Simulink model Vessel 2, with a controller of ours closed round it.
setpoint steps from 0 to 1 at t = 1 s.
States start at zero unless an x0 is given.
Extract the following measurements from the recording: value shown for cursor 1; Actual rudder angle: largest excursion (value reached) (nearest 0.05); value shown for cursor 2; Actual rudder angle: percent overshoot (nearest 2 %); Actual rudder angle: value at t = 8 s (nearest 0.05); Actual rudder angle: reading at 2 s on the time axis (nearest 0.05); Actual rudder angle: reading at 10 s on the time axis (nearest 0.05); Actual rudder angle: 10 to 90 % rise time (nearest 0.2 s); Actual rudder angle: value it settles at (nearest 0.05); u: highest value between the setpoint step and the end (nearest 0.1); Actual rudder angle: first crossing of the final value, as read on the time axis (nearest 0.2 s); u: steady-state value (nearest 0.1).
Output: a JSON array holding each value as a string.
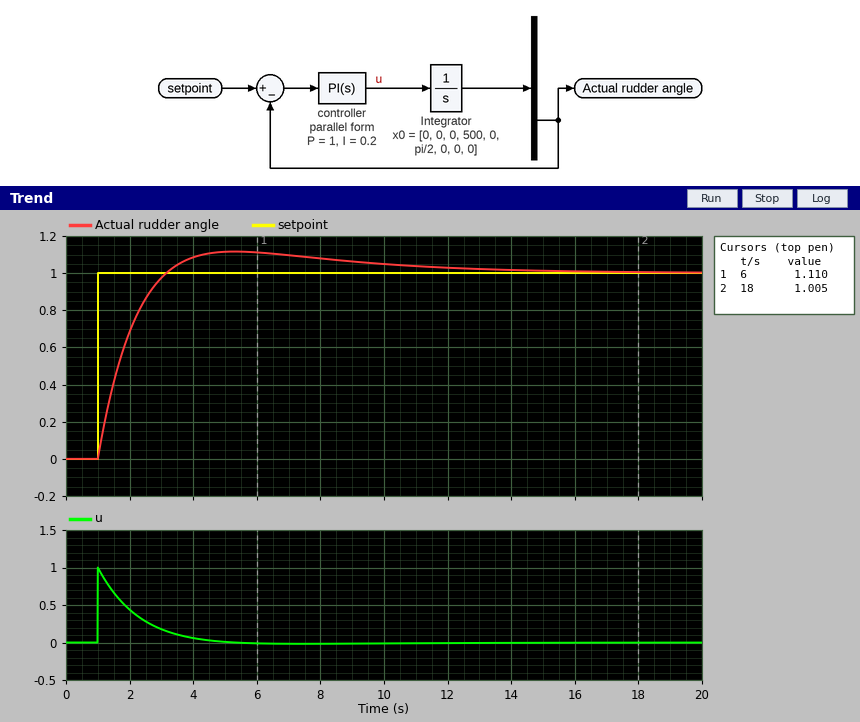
["1.110", "1.10", "1.005", "12 %", "1.10", "0.70", "1.05", "1.6 s", "1.00", "1.0", "3.2 s", "0.0"]
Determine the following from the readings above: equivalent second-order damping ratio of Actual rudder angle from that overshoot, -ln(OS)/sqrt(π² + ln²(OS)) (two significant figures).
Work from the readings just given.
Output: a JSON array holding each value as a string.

["0.56"]
